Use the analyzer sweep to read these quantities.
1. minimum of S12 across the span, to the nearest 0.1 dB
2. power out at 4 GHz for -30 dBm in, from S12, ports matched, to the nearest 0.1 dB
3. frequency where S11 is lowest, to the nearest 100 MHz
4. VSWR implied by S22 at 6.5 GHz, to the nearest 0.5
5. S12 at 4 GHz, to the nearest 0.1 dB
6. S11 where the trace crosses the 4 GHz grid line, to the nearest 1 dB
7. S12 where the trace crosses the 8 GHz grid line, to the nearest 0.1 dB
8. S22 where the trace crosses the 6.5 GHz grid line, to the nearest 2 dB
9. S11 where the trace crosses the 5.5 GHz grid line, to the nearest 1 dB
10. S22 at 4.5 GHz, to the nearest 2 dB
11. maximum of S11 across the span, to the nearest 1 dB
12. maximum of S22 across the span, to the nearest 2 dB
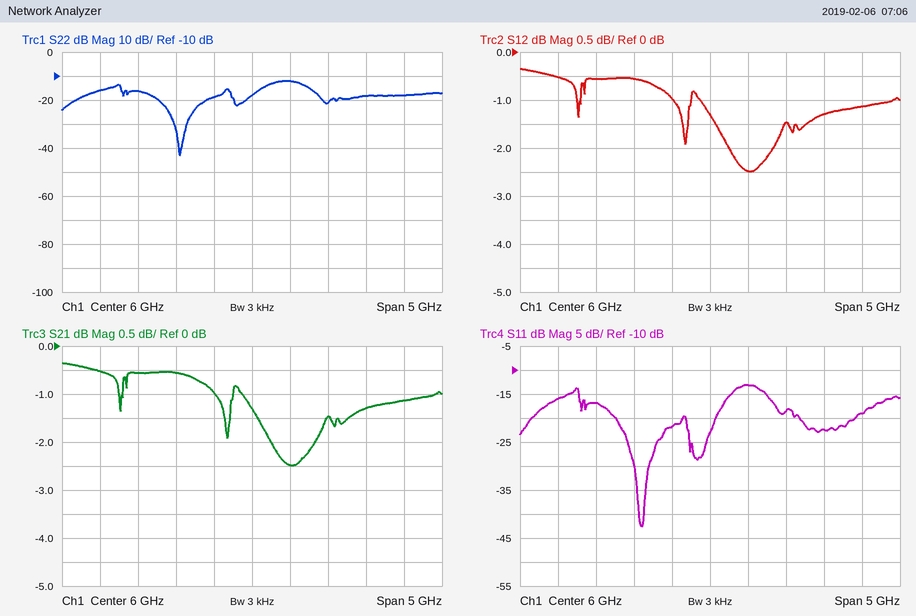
-2.5 dB
-30.5 dBm
5.1 GHz
1.5
-0.5 dB
-16 dB
-1.1 dB
-12 dB
-22 dB
-16 dB
-13 dB
-12 dB
